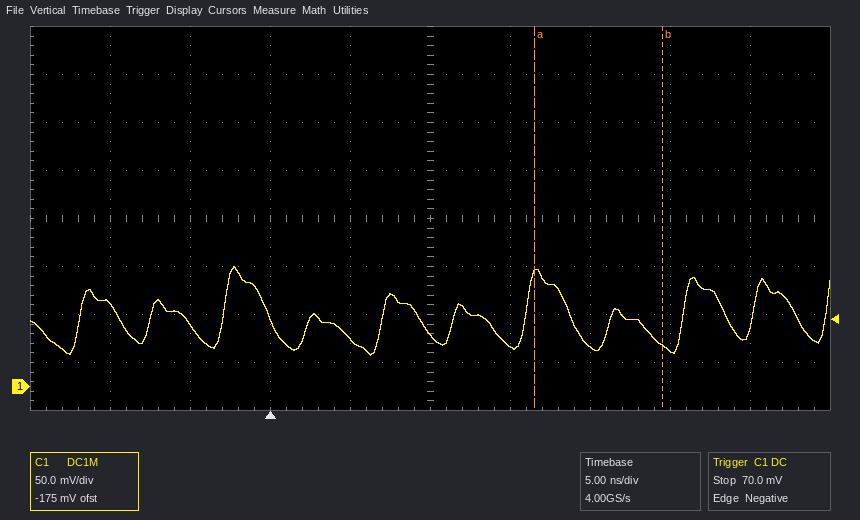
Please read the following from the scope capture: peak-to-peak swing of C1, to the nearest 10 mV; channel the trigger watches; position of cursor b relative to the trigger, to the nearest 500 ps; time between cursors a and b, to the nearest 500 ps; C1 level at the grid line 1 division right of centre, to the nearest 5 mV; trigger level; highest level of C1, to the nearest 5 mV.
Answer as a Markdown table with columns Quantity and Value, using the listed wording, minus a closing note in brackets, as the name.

| Quantity | Value |
|---|---|
| peak-to-peak swing of C1, to the nearest 10 mV | 90 mV |
| channel the trigger watches | C1 |
| position of cursor b relative to the trigger, to the nearest 500 ps | +24.5 ns |
| time between cursors a and b, to the nearest 500 ps | 8.0 ns |
| C1 level at the grid line 1 division right of centre, to the nearest 5 mV | 40 mV |
| trigger level | 70.0 mV |
| highest level of C1, to the nearest 5 mV | 125 mV |
